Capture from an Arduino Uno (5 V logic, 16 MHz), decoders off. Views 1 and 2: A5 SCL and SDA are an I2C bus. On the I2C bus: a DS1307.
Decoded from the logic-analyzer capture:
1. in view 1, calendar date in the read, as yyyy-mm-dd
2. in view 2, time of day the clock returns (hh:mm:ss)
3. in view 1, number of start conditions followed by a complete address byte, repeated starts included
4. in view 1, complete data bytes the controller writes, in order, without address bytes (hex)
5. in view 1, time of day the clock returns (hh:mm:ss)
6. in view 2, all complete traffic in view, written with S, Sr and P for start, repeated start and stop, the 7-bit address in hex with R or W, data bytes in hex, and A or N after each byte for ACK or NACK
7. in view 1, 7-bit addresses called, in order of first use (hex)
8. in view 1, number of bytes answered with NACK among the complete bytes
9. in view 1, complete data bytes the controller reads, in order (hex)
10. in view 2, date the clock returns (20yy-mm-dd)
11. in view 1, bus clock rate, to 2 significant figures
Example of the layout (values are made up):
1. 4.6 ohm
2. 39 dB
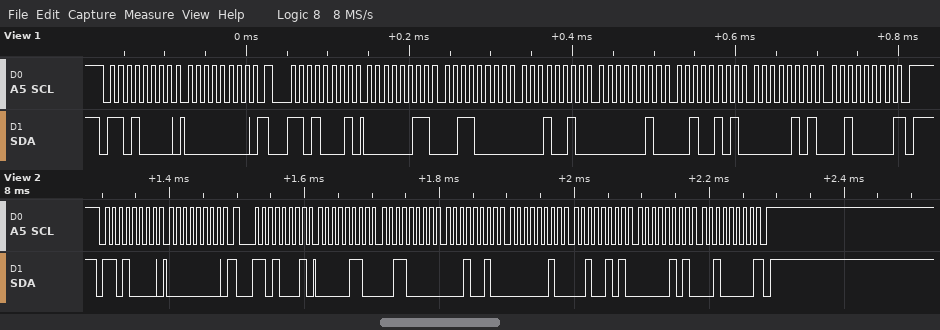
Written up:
1. 2020-05-25
2. 12:30:06
3. 2
4. 00
5. 12:30:03
6. S 68W A 00 A Sr 68R A 06 A 30 A 12 A 02 A 25 A 05 A 20 N P
7. 0x68
8. 1
9. 03 30 12 02 25 05 20
10. 2020-05-25
11. 100 kHz
